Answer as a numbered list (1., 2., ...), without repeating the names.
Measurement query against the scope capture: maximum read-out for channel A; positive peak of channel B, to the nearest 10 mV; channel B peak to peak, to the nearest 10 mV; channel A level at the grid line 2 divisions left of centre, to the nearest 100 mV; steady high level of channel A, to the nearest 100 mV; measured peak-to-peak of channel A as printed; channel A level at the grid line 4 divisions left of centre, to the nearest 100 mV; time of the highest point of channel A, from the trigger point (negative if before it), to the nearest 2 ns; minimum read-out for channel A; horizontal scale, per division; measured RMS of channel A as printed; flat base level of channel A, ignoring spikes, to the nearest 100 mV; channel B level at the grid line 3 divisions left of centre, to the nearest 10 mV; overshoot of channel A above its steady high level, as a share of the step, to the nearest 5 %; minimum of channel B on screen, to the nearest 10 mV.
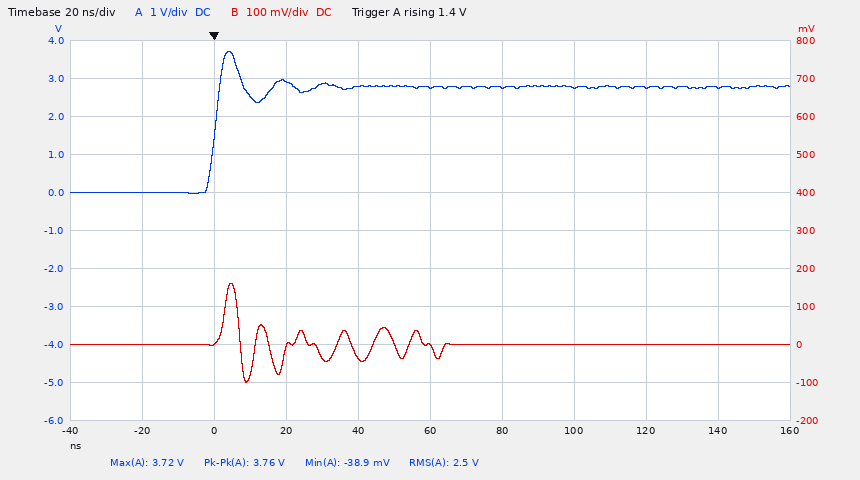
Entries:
1. 3.72 V
2. 160 mV
3. 260 mV
4. 2.9 V
5. 2.8 V
6. 3.76 V
7. 0.0 V
8. +4 ns
9. -38.9 mV
10. 20 ns
11. 2.5 V
12. 0.0 V
13. 0 mV
14. 35 %
15. -100 mV
